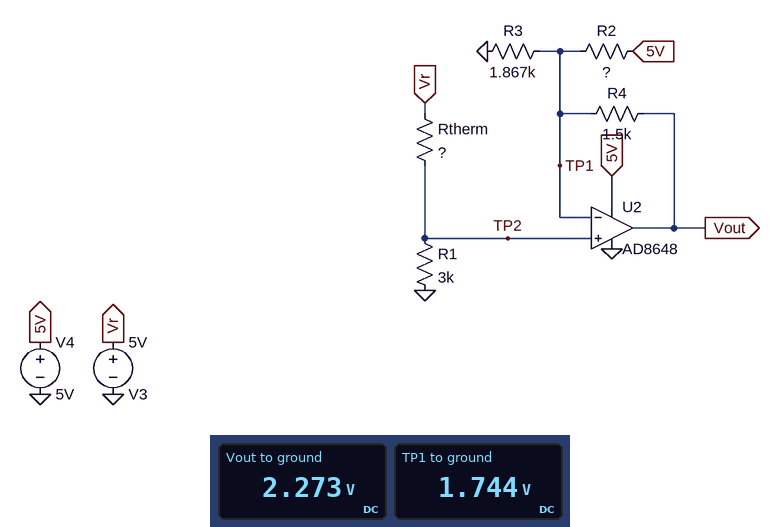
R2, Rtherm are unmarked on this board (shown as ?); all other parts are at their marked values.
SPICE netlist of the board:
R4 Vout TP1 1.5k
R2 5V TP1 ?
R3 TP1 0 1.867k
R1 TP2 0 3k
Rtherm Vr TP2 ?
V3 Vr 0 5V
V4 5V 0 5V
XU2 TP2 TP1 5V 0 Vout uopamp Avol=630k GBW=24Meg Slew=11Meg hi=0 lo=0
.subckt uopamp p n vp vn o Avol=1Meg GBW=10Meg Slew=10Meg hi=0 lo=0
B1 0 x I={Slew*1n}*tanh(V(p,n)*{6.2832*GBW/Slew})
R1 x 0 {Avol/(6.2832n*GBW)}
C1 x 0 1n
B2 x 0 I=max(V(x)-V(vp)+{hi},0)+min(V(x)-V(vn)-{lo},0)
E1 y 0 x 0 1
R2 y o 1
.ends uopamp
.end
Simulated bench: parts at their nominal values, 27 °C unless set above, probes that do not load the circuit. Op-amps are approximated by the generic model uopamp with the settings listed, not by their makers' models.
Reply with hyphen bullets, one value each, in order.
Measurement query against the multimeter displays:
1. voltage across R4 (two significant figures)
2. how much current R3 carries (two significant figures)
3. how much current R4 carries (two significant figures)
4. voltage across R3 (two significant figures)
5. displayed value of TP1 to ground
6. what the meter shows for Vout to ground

- 530 mV
- 930 µA
- 350 µA
- 1.7 V
- 1.744 V
- 2.273 V
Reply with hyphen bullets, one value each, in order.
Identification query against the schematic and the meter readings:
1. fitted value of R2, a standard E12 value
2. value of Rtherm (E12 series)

- 5.6 kΩ
- 5.6 kΩ
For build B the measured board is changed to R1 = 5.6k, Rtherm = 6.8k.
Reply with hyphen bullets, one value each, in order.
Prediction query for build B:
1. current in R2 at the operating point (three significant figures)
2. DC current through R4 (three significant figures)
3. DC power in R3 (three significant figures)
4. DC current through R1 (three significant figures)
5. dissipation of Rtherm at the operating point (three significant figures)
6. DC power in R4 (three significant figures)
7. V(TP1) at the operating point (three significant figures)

- 490 µA
- 720 µA
- 2.73 mW
- 403 µA
- 1.11 mW
- 777 µW
- 2.26 V
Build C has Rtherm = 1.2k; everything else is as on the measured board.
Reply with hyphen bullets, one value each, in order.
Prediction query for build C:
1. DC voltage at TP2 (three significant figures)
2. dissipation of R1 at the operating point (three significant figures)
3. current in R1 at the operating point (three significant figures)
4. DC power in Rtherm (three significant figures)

- 3.57 V
- 4.25 mW
- 1.19 mA
- 1.70 mW
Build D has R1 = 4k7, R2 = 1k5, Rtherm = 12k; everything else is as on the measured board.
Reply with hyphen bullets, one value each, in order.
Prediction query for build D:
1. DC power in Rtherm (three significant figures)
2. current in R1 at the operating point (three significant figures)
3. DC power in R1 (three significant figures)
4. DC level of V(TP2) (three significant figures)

- 1.08 mW
- 299 µA
- 421 µW
- 1.41 V
